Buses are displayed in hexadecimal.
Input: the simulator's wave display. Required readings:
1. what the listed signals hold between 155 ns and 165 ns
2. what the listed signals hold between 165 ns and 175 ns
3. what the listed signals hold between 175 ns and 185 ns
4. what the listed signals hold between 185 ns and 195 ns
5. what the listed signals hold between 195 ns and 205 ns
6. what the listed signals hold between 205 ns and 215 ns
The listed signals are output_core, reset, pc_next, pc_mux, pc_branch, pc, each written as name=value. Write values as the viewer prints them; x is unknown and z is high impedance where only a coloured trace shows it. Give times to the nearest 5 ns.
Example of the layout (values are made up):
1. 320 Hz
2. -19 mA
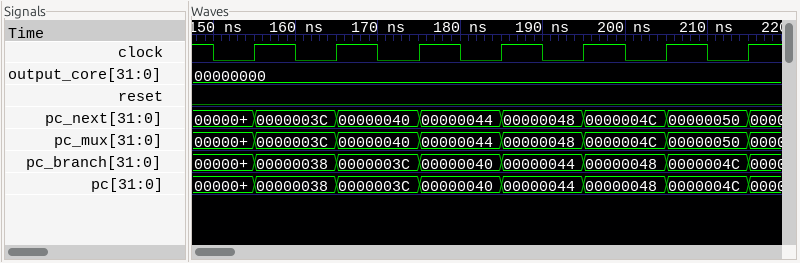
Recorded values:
1. output_core=00000000, reset=0, pc_next=0000003C, pc_mux=0000003C, pc_branch=00000038, pc=00000038
2. output_core=00000000, reset=0, pc_next=00000040, pc_mux=00000040, pc_branch=0000003C, pc=0000003C
3. output_core=00000000, reset=0, pc_next=00000044, pc_mux=00000044, pc_branch=00000040, pc=00000040
4. output_core=00000000, reset=0, pc_next=00000048, pc_mux=00000048, pc_branch=00000044, pc=00000044
5. output_core=00000000, reset=0, pc_next=0000004C, pc_mux=0000004C, pc_branch=00000048, pc=00000048
6. output_core=00000000, reset=0, pc_next=00000050, pc_mux=00000050, pc_branch=0000004C, pc=0000004C
